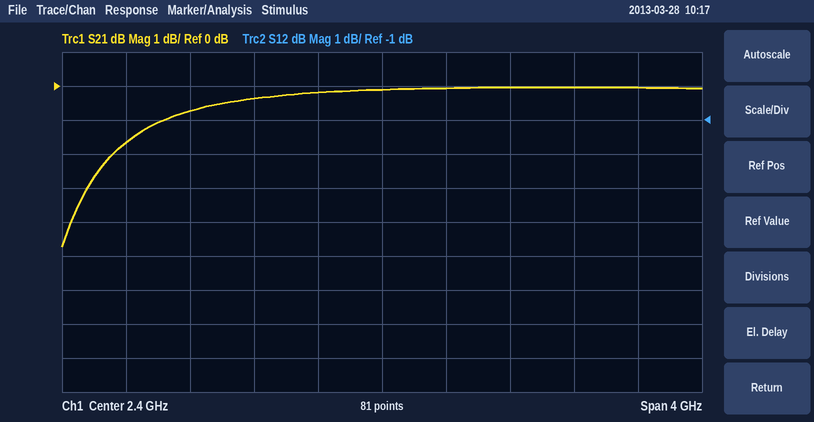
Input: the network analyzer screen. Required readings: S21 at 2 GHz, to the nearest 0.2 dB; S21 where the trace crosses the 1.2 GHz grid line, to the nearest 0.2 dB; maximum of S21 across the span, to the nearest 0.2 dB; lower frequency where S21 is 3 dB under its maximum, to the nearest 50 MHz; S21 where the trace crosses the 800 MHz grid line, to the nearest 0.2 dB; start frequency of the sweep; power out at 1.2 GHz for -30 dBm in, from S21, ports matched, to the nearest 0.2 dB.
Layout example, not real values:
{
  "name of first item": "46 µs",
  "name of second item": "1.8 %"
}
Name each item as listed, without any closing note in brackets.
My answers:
{
  "S21 at 2 GHz, to the nearest 0.2 dB": "-0.2 dB",
  "S21 where the trace crosses the 1.2 GHz grid line, to the nearest 0.2 dB": "-0.8 dB",
  "maximum of S21 across the span, to the nearest 0.2 dB": "0.0 dB",
  "lower frequency where S21 is 3 dB under its maximum, to the nearest 50 MHz": "550 MHz",
  "S21 where the trace crosses the 800 MHz grid line, to the nearest 0.2 dB": "-1.6 dB",
  "start frequency of the sweep": "400 MHz",
  "power out at 1.2 GHz for -30 dBm in, from S21, ports matched, to the nearest 0.2 dB": "-30.8 dBm"
}
